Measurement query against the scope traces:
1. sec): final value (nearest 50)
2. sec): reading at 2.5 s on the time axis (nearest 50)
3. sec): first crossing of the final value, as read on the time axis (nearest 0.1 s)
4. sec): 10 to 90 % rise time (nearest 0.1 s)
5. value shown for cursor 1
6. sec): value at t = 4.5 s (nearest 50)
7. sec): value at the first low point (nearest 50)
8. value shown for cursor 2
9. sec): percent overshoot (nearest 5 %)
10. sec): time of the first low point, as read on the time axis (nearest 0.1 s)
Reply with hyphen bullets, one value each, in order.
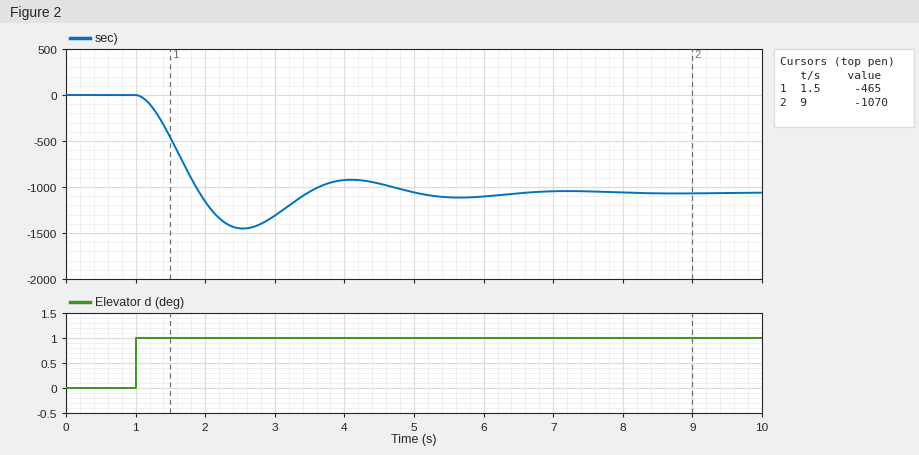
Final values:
- -1050
- -1450
- 1.9 s
- 0.6 s
- -465
- -950
- -1450
- -1070
- 35 %
- 2.5 s
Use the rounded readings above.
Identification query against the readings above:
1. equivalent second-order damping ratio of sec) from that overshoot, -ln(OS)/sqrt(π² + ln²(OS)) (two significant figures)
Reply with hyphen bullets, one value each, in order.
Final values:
- 0.32
